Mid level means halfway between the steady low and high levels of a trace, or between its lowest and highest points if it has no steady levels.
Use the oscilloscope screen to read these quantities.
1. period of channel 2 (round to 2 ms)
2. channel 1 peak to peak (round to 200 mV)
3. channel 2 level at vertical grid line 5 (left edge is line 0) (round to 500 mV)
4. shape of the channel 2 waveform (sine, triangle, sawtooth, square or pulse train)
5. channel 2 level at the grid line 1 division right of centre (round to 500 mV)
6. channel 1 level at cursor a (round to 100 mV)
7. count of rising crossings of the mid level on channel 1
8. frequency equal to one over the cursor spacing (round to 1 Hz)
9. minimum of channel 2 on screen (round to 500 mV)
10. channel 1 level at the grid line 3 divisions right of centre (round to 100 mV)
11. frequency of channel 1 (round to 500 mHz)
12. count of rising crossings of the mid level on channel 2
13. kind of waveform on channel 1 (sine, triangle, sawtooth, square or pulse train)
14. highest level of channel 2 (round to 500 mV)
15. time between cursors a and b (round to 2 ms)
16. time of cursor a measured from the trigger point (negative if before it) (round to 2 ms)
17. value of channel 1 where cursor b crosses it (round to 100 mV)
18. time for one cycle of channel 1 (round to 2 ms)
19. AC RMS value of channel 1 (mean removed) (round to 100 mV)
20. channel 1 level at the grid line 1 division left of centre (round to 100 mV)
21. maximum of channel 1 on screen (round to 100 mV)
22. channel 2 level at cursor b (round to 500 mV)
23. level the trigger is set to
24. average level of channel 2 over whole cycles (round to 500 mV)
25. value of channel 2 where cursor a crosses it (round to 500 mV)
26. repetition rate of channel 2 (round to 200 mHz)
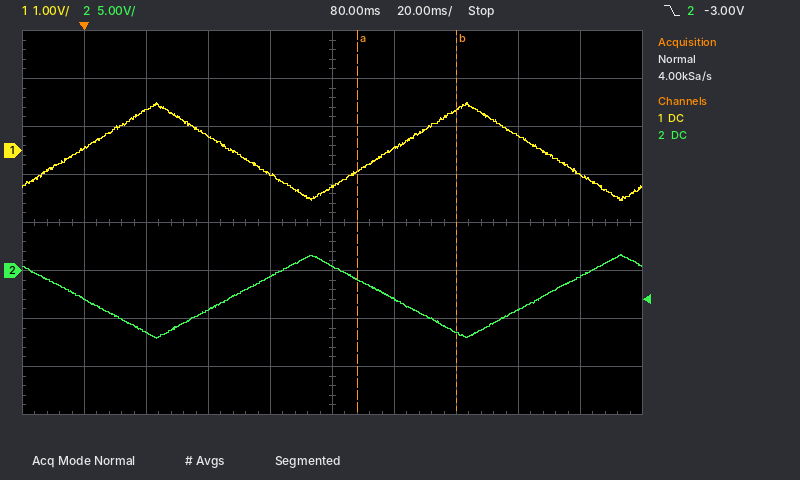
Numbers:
100 ms
2.0 V
500 mV
triangle
-3.0 V
-400 mV
2
31 Hz
-7.0 V
300 mV
10.0 Hz
2
triangle
1.5 V
32 ms
+88 ms
900 mV
100 ms
600 mV
-500 mV
1.0 V
-6.5 V
-3.00 V
-2.5 V
-1.0 V
10.0 Hz
